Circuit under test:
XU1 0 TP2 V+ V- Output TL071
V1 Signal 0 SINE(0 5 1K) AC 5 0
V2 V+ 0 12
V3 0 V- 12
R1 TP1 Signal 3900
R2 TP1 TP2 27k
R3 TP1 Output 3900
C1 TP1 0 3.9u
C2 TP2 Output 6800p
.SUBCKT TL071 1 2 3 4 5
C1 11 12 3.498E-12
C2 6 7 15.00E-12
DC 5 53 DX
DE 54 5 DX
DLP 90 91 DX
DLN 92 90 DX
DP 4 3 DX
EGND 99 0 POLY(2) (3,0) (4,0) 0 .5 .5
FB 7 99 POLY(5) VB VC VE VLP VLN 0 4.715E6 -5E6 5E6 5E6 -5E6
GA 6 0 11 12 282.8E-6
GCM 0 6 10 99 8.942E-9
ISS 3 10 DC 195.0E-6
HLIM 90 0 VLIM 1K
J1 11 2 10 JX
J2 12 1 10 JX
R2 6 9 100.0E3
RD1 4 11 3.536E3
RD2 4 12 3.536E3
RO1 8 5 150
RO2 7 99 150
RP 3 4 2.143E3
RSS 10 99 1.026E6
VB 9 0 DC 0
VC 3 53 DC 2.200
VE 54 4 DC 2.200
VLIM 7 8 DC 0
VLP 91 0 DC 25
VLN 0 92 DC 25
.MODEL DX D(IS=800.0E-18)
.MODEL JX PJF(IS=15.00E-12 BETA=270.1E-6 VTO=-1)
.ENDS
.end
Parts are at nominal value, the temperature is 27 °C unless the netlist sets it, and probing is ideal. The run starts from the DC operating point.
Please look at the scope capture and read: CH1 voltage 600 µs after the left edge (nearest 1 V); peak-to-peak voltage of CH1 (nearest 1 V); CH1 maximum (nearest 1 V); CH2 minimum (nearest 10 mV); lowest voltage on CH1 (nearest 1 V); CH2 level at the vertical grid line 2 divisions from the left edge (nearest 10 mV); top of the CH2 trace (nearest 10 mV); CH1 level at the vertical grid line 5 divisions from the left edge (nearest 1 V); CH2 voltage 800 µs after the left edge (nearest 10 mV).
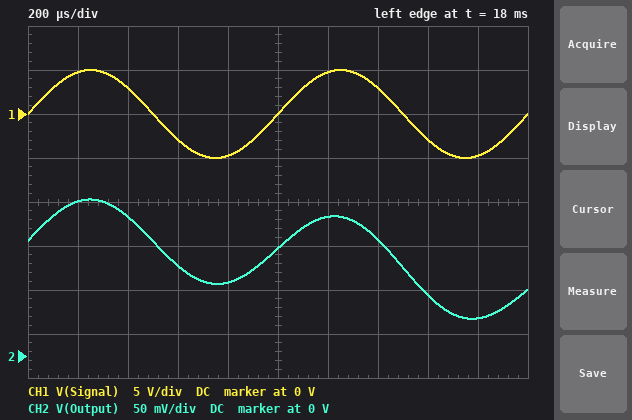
-3 V
10 V
5 V
40 mV
-5 V
160 mV
180 mV
0 V
80 mV
